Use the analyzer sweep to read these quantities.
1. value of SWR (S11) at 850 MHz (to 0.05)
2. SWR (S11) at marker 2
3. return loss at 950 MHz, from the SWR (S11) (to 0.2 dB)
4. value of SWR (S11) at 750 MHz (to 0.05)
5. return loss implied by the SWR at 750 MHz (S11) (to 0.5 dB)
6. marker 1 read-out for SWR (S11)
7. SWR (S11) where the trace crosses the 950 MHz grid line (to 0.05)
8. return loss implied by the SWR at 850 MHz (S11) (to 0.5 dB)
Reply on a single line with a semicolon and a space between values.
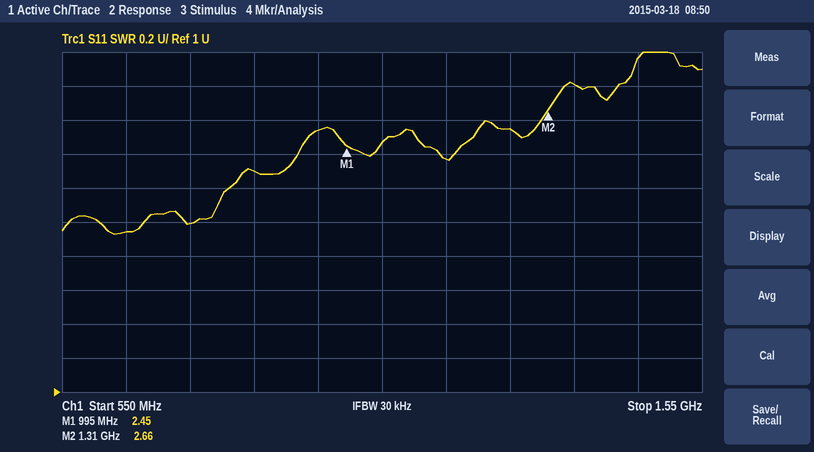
2.30; 2.66; 7.2 dB; 2.00; 9.5 dB; 2.45; 2.55; 8.0 dB
